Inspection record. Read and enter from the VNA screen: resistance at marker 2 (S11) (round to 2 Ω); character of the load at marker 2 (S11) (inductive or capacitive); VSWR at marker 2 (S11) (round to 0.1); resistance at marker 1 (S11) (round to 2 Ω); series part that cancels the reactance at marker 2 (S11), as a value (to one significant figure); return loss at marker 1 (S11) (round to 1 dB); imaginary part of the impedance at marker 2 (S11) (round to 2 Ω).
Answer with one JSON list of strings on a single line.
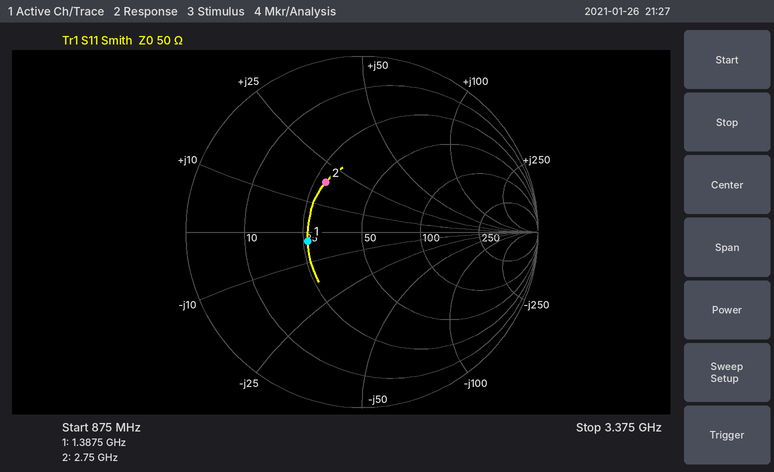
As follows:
["28 Ω", "inductive", "2.1", "26 Ω", "3 pF", "10 dB", "+18 Ω"]
